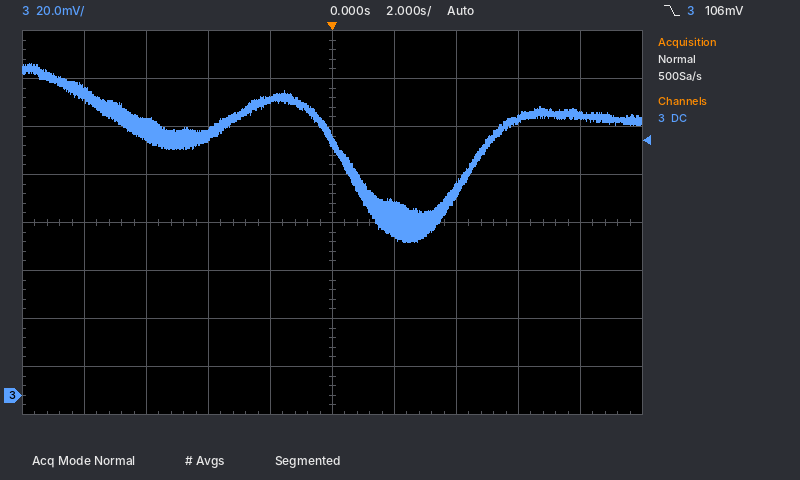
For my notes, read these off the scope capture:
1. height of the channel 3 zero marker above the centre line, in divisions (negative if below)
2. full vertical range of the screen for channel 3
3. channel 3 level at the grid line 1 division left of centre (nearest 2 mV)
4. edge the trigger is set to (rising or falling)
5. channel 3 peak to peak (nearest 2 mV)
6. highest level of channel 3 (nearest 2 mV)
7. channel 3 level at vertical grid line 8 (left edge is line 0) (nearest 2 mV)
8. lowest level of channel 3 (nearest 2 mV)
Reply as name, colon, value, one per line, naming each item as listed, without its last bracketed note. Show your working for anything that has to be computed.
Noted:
height of the channel 3 zero marker above the centre line, in divisions: -3.6 div
full vertical range of the screen for channel 3: 160 mV
channel 3 level at the grid line 1 division left of centre: 124 mV
edge the trigger is set to: falling
channel 3 peak to peak: 138 mV − (64 mV) = 74 mV
highest level of channel 3: 138 mV
channel 3 level at vertical grid line 8 (left edge is line 0): 116 mV
lowest level of channel 3: 64 mV
